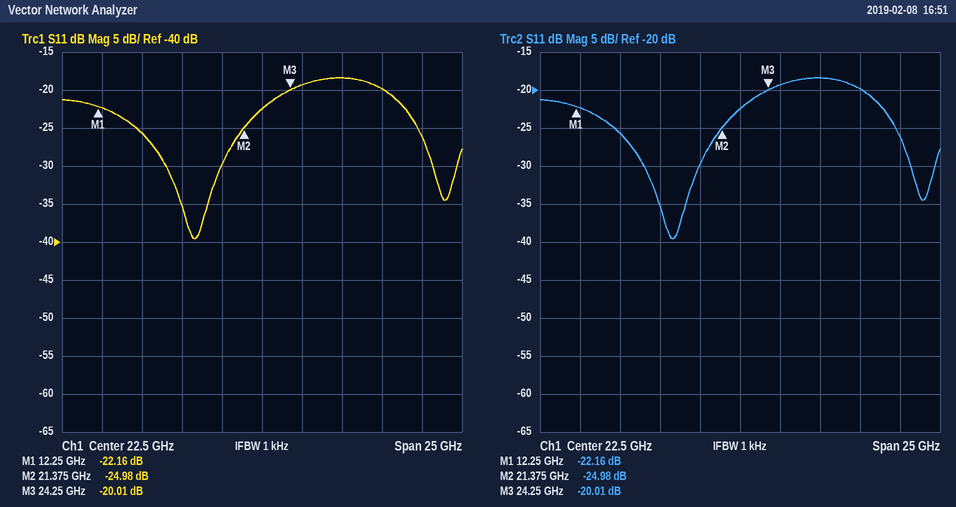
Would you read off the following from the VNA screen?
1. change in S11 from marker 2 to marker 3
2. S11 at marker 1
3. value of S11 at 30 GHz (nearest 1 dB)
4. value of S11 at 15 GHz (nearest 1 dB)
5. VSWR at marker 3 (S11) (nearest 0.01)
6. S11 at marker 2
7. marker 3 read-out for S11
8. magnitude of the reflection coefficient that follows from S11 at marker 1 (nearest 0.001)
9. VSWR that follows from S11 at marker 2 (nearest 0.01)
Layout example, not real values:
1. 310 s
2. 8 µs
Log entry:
1. 4.97 dB
2. -22.16 dB
3. -20 dB
4. -26 dB
5. 1.22
6. -24.98 dB
7. -20.01 dB
8. 0.078
9. 1.12
